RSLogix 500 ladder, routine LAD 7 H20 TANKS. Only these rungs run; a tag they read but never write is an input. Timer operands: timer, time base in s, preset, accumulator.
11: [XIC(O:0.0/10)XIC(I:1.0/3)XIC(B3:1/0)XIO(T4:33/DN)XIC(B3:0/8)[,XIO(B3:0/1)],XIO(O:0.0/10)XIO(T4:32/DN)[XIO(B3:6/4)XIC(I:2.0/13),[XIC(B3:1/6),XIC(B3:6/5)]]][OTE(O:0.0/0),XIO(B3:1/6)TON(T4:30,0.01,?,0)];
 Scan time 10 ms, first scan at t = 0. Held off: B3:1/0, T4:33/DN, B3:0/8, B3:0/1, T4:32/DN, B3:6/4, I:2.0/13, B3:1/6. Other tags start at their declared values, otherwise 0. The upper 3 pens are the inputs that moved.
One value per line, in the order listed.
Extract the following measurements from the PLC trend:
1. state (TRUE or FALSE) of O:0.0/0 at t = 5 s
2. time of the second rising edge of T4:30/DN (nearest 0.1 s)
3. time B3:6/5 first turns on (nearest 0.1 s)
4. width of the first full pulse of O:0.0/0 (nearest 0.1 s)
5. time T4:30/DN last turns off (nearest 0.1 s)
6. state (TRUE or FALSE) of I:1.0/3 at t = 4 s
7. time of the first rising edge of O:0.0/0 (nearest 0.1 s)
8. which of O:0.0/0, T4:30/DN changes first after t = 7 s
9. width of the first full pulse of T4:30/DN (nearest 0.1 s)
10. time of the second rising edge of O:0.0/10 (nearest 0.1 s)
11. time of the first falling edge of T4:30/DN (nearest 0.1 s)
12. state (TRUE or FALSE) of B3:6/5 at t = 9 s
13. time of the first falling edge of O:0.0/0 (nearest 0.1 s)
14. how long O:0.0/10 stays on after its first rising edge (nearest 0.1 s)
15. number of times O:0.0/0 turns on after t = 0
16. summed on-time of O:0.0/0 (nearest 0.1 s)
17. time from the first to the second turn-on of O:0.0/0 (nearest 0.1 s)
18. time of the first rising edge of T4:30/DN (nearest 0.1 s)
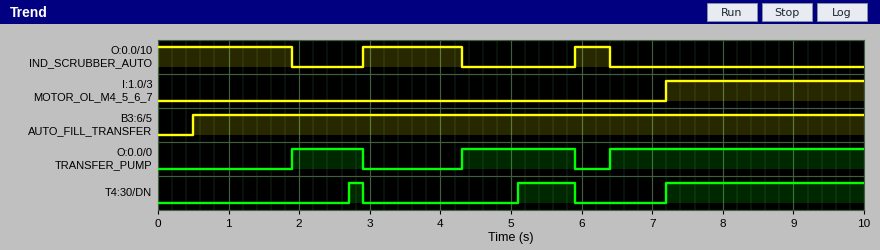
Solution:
TRUE
5.1 s
0.5 s
1.0 s
5.9 s
FALSE
1.9 s
T4:30/DN
0.2 s
5.9 s
2.9 s
TRUE
2.9 s
1.4 s
3
6.2 s
2.4 s
2.7 s
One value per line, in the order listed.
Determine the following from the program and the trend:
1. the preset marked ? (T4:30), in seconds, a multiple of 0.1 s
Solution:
0.8 s
